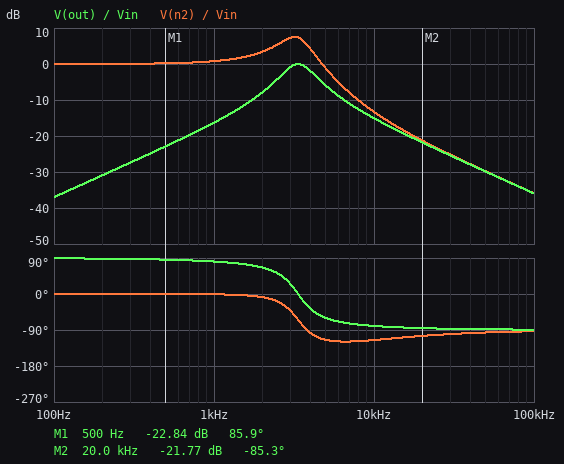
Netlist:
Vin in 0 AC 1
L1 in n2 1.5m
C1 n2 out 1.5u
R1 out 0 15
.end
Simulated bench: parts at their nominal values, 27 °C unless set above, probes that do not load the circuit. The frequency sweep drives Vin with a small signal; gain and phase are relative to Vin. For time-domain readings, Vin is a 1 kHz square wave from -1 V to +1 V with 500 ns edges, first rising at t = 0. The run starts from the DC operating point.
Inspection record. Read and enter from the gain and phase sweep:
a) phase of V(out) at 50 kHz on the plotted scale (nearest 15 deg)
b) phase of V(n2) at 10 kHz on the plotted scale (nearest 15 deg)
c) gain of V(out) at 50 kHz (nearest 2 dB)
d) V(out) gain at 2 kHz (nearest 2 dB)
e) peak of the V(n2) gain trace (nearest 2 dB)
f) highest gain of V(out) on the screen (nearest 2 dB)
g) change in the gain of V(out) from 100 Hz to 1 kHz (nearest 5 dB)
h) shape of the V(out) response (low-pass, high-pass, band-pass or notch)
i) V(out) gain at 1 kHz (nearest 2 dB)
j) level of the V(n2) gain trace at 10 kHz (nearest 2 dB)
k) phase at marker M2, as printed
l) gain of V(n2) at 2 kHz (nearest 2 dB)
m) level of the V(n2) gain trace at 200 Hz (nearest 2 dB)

-90 deg
-120 deg
-30 dB
-8 dB
8 dB
0 dB
20 dB
band-pass
-16 dB
-14 dB
-85.3 deg
4 dB
0 dB
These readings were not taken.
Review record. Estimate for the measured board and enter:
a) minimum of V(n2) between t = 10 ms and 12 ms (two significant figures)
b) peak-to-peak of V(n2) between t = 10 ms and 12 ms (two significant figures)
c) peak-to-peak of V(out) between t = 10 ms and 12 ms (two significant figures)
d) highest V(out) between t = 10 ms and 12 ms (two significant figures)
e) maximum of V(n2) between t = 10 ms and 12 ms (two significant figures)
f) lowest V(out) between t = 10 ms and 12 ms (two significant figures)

-2.1 V
4.2 V
1.5 V
740 mV
2.1 V
-740 mV
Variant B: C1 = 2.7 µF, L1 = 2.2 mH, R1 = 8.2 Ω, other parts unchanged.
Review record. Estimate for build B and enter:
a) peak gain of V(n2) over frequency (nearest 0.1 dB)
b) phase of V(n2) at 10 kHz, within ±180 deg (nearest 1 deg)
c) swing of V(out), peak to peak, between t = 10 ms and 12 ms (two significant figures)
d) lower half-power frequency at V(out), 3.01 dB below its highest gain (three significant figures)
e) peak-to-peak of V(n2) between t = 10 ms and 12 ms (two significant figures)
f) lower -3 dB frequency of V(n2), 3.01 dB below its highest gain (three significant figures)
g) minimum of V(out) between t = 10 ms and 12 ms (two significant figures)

11.3 dB
-122 deg
670 mV
1.79 kHz
3.9 V
1.70 kHz
-330 mV
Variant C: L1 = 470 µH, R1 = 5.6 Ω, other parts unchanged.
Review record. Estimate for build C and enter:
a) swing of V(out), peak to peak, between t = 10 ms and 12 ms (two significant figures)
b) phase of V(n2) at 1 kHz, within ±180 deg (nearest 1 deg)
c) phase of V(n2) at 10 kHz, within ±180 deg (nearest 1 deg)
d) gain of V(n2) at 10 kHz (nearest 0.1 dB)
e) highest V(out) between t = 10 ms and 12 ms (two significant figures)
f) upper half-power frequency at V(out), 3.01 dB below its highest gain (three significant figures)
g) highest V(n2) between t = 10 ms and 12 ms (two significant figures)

960 mV
0 deg
-136 deg
-4.3 dB
480 mV
7.02 kHz
2.2 V
